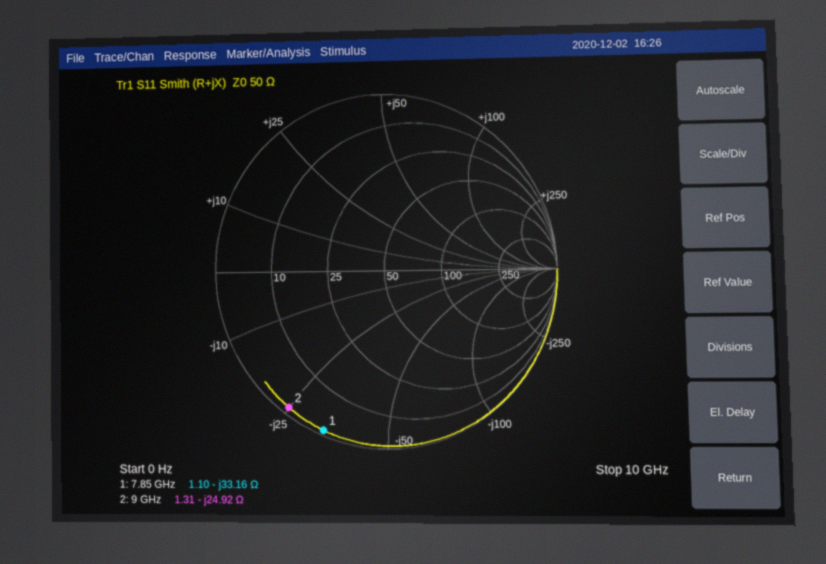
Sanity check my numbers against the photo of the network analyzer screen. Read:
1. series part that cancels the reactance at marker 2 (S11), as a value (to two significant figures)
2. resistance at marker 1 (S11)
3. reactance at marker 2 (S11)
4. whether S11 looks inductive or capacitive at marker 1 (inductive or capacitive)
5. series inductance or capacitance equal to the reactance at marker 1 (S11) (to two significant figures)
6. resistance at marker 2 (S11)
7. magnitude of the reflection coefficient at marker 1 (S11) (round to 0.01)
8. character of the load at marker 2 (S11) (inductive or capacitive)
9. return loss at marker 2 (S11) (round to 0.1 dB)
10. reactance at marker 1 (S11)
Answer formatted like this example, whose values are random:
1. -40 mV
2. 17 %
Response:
1. 440 pH
2. 1.10 Ω
3. -24.92 Ω
4. capacitive
5. 610 fF
6. 1.31 Ω
7. 0.97
8. capacitive
9. 0.4 dB
10. -33.16 Ω
